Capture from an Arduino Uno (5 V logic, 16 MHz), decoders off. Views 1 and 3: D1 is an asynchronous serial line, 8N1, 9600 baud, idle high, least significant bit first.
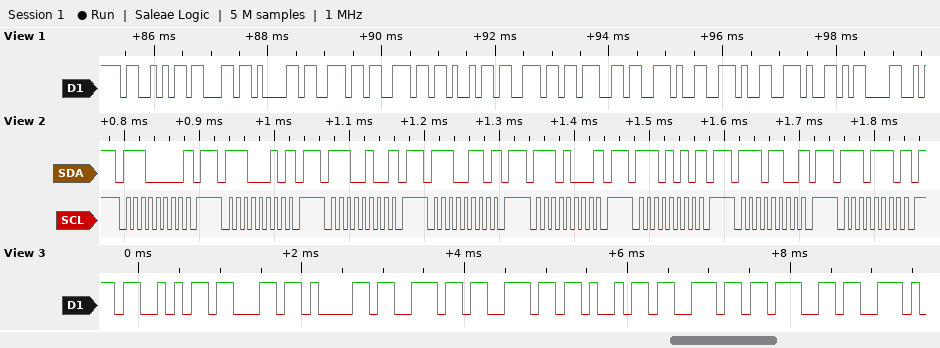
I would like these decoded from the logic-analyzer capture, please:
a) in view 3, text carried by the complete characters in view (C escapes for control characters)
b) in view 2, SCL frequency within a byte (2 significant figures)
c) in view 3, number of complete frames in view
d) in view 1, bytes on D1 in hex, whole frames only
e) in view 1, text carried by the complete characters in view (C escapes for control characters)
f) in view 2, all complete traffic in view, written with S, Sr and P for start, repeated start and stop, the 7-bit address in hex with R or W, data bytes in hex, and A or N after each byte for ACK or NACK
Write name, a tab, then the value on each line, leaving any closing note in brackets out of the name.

in view 3, text carried by the complete characters in view	"Scanning"
in view 2, SCL frequency within a byte	100 kHz
in view 3, number of complete frames in view	8
in view 1, bytes on D1 in hex, whole frames only	53 63 61 6E 6E 69 6E 67 2E 2E 2E 0D
in view 1, text carried by the complete characters in view	"Scanning...\r"
in view 2, all complete traffic in view, written with S, Sr and P for start, repeated start and stop, the 7-bit address in hex with R or W, data bytes in hex, and A or N after each byte for ACK or NACK	S 70W N P S 71W N P S 72W N P S 73W N P S 74W N P S 75W N P S 76W N P S 77W N P
